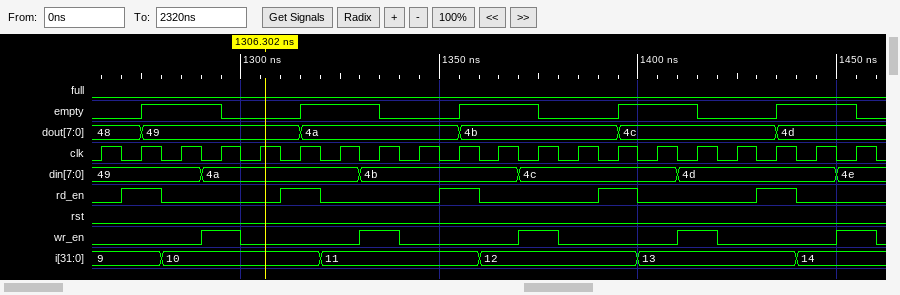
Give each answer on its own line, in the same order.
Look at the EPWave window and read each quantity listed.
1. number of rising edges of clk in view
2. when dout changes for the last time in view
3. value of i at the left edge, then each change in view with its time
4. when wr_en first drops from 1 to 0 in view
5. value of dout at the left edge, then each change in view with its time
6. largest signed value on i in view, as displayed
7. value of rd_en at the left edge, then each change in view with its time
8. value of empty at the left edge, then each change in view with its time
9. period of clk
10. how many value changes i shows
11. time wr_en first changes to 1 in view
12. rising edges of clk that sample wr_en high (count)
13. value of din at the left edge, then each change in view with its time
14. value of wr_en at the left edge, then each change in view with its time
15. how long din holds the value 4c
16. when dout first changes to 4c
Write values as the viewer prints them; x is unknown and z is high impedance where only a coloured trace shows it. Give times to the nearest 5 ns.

20
1435 ns
9, 10 at 1280 ns, 11 at 1320 ns, 12 at 1360 ns, 13 at 1400 ns, 14 at 1440 ns
1300 ns
48, 49 at 1275 ns, 4a at 1315 ns, 4b at 1355 ns, 4c at 1395 ns, 4d at 1435 ns
14
0, 1 at 1270 ns, 0 at 1280 ns, 1 at 1310 ns, 0 at 1320 ns, 1 at 1350 ns, 0 at 1360 ns, 1 at 1390 ns, 0 at 1400 ns, 1 at 1430 ns, 0 at 1440 ns
0, 1 at 1275 ns, 0 at 1295 ns, 1 at 1315 ns, 0 at 1335 ns, 1 at 1355 ns, 0 at 1375 ns, 1 at 1395 ns, 0 at 1415 ns, 1 at 1435 ns, 0 at 1455 ns
10 ns
5
1290 ns
5
49, 4a at 1290 ns, 4b at 1330 ns, 4c at 1370 ns, 4d at 1410 ns, 4e at 1450 ns
0, 1 at 1290 ns, 0 at 1300 ns, 1 at 1330 ns, 0 at 1340 ns, 1 at 1370 ns, 0 at 1380 ns, 1 at 1410 ns, 0 at 1420 ns, 1 at 1450 ns, 0 at 1460 ns
40 ns
1395 ns
